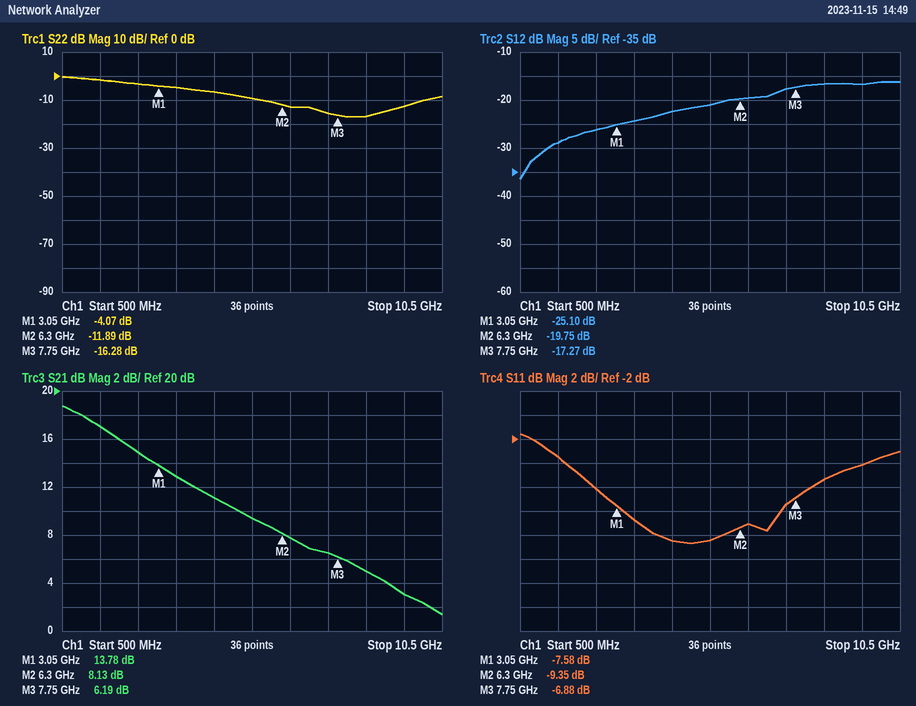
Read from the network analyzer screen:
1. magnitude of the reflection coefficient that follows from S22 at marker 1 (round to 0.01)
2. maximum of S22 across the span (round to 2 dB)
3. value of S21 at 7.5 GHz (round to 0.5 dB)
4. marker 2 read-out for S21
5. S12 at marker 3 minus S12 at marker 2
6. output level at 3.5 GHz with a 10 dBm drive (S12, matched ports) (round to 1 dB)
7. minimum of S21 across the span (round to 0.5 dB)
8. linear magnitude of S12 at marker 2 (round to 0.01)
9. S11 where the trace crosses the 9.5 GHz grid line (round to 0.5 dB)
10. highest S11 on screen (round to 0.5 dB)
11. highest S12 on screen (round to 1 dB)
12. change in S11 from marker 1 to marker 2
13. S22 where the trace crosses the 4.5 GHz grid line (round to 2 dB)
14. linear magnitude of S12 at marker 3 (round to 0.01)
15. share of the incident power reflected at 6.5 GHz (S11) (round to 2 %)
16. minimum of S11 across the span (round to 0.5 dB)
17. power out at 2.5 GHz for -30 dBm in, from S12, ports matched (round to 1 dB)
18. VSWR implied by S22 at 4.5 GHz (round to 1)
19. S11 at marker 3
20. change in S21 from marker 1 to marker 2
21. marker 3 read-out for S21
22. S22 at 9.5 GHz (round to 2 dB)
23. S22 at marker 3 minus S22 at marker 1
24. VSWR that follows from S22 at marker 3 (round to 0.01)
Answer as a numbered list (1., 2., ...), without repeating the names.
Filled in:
1. 0.63
2. 0 dB
3. 6.5 dB
4. 8.13 dB
5. 2.48 dB
6. -14 dBm
7. 1.5 dB
8. 0.10
9. -4.0 dB
10. -1.5 dB
11. -16 dB
12. -1.77 dB
13. -6 dB
14. 0.14
15. 12 %
16. -10.5 dB
17. -56 dBm
18. 3
19. -6.88 dB
20. -5.65 dB
21. 6.19 dB
22. -12 dB
23. -12.21 dB
24. 1.36
